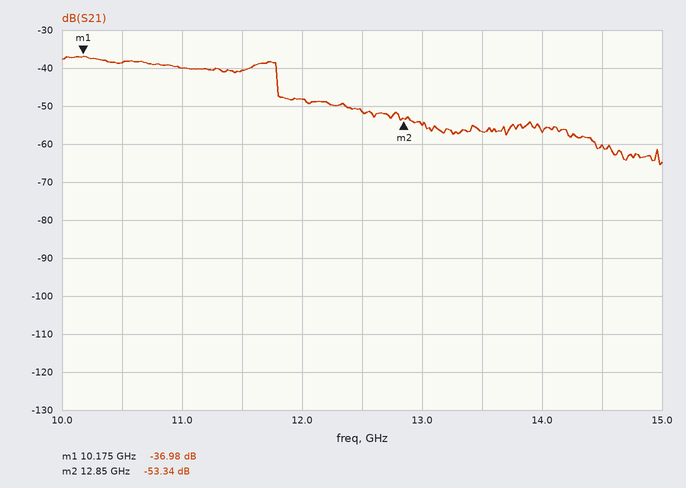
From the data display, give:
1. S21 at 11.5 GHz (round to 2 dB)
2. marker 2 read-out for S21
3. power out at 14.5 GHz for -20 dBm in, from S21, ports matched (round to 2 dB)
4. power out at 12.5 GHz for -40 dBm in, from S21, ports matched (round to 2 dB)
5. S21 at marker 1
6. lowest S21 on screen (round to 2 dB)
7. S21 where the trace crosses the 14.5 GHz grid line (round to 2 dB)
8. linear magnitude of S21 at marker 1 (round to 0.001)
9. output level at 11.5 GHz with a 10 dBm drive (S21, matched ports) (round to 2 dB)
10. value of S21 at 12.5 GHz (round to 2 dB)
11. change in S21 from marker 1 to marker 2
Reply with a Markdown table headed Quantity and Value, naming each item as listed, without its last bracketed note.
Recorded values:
| Quantity | Value |
|---|---|
| S21 at 11.5 GHz | -40 dB |
| marker 2 read-out for S21 | -53.34 dB |
| power out at 14.5 GHz for -20 dBm in, from S21, ports matched | -80 dBm |
| power out at 12.5 GHz for -40 dBm in, from S21, ports matched | -92 dBm |
| S21 at marker 1 | -36.98 dB |
| lowest S21 on screen | -66 dB |
| S21 where the trace crosses the 14.5 GHz grid line | -60 dB |
| linear magnitude of S21 at marker 1 | 0.014 |
| output level at 11.5 GHz with a 10 dBm drive (S21, matched ports) | -30 dBm |
| value of S21 at 12.5 GHz | -52 dB |
| change in S21 from marker 1 to marker 2 | -16.36 dB |
